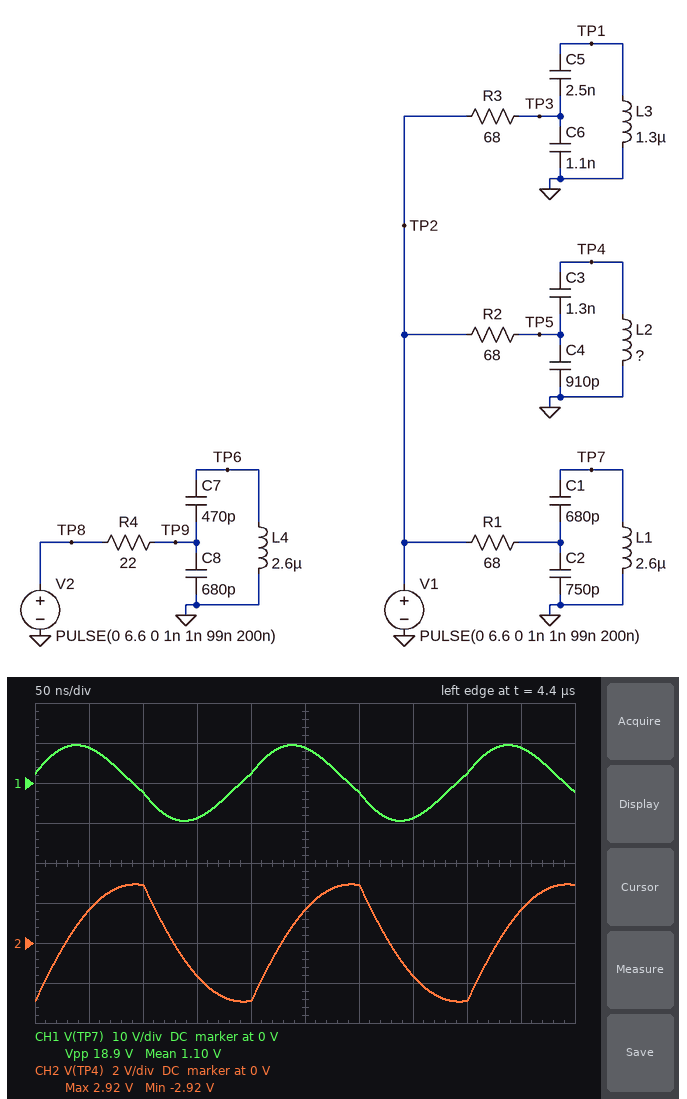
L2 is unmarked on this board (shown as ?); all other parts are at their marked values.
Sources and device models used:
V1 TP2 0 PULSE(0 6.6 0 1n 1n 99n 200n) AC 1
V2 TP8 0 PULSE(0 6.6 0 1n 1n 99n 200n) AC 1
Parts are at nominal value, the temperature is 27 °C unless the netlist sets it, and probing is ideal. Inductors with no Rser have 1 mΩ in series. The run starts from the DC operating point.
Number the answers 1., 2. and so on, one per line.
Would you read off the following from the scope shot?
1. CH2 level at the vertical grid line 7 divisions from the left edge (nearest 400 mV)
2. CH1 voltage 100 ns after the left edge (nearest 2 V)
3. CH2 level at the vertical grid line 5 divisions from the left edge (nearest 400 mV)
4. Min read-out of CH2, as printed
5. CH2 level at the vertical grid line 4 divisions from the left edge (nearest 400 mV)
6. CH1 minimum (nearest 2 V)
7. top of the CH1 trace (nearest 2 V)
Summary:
1. -1.6 V
2. -2 V
3. 1.6 V
4. -2.92 V
5. -2.8 V
6. -10 V
7. 10 V
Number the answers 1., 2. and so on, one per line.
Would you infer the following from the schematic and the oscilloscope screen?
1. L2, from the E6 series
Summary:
1. 4.7 µH
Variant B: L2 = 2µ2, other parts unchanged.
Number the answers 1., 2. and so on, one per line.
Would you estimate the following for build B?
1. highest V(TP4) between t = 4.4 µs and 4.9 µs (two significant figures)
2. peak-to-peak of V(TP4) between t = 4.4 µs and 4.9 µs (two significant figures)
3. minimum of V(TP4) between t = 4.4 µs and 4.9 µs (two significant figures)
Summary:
1. 5.8 V
2. 12 V
3. -5.8 V
